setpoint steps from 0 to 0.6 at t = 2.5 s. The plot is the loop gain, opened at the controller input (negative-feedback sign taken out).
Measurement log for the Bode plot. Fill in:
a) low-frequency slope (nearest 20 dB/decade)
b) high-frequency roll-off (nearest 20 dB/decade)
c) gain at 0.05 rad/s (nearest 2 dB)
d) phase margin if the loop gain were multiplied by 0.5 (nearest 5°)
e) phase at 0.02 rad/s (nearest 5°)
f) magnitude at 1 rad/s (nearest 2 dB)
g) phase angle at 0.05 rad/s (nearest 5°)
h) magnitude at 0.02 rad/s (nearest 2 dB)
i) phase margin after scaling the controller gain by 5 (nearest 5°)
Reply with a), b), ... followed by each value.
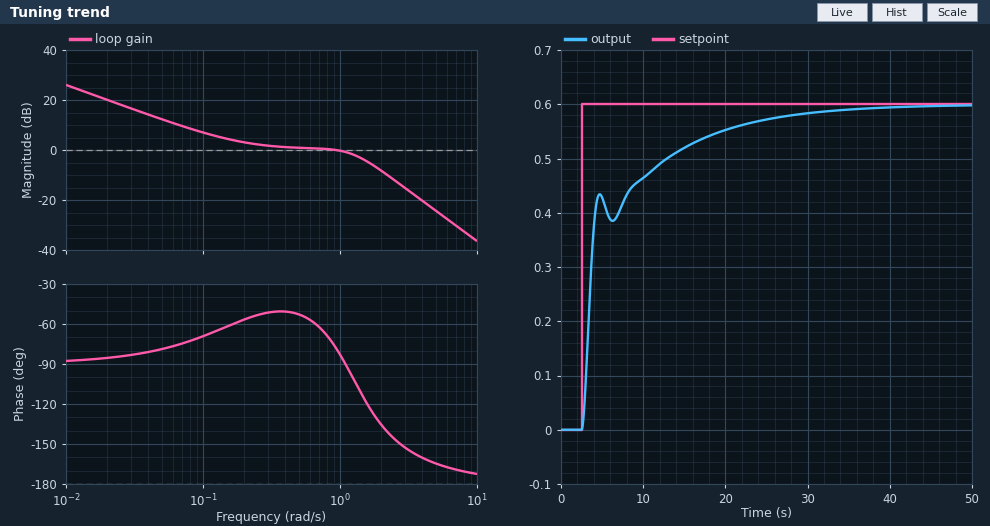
a) -20 dB/decade
b) -40 dB/decade
c) 12 dB
d) 115°
e) -85°
f) 0 dB
g) -80°
h) 20 dB
i) 30°
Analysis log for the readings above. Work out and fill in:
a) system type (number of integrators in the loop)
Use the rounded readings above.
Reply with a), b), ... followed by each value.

a) 1
